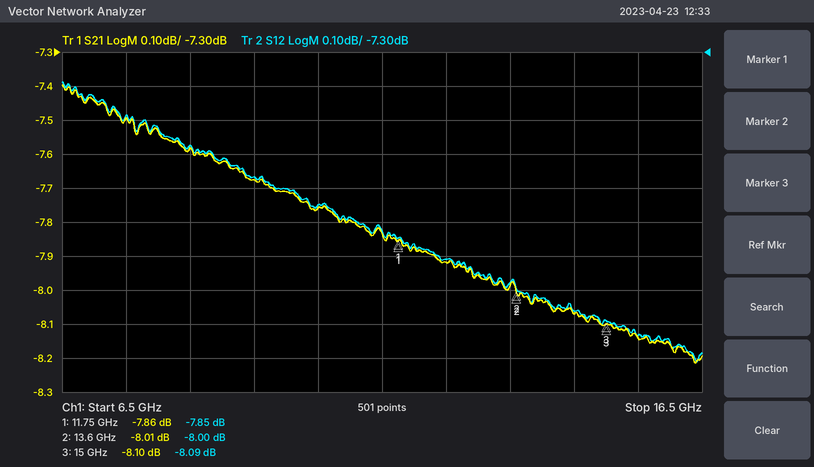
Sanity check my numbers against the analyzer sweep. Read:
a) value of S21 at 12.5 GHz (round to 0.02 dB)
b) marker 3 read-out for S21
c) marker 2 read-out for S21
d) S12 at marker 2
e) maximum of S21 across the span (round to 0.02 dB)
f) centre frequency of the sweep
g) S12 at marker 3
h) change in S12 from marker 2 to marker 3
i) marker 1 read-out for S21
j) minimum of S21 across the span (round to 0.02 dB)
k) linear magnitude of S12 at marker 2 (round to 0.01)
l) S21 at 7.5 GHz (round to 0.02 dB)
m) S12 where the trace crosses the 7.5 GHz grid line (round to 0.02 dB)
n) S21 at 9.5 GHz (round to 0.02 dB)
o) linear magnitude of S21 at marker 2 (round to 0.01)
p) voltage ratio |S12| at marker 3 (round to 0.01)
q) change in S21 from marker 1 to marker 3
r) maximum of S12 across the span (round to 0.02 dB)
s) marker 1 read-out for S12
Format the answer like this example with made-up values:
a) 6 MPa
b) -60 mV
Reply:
a) -7.92 dB
b) -8.10 dB
c) -8.01 dB
d) -8.00 dB
e) -7.40 dB
f) 11.5 GHz
g) -8.09 dB
h) -0.09 dB
i) -7.86 dB
j) -8.22 dB
k) 0.40
l) -7.50 dB
m) -7.48 dB
n) -7.68 dB
o) 0.40
p) 0.39
q) -0.24 dB
r) -7.38 dB
s) -7.85 dB
